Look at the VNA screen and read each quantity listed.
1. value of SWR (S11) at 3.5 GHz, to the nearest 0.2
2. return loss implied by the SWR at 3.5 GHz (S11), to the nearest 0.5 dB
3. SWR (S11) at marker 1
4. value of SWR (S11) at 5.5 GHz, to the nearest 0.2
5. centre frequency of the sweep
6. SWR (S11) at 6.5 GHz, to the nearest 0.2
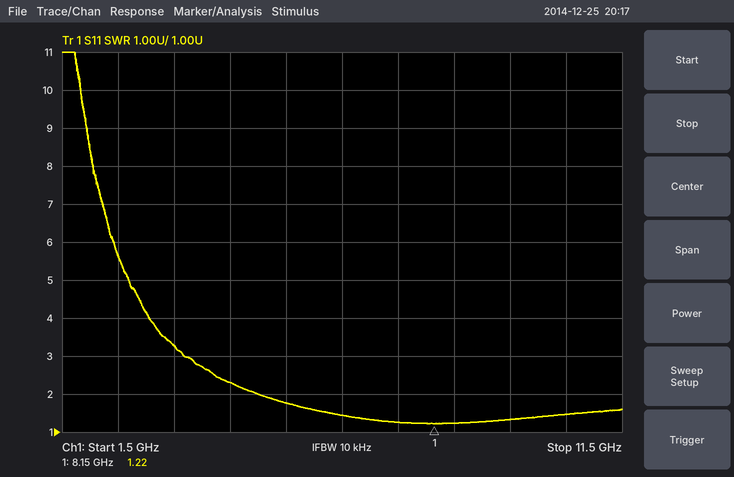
3.2
5.5 dB
1.22
1.8
6.5 GHz
1.4
